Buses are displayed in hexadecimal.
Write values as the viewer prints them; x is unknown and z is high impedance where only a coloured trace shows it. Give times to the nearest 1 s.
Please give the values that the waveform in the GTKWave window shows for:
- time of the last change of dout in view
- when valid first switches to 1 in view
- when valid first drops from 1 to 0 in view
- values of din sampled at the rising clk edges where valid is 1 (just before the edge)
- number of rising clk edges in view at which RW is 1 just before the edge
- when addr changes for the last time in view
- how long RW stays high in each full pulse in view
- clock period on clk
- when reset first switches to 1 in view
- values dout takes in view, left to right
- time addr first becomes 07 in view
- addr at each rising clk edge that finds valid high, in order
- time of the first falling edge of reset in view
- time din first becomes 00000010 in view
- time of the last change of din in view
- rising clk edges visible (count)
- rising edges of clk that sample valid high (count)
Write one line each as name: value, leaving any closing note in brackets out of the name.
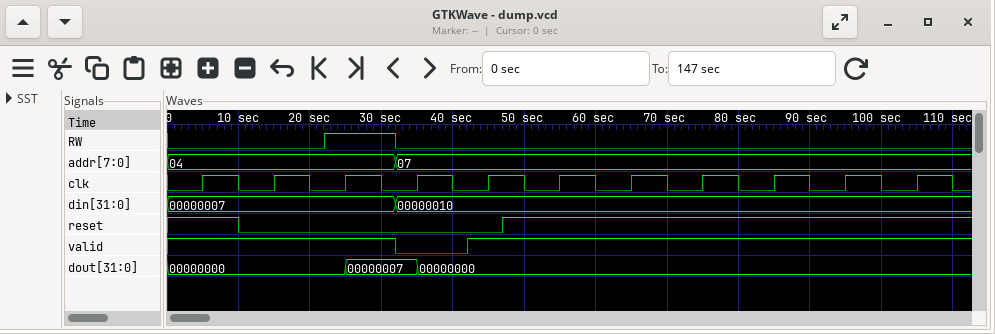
time of the last change of dout in view: 35 s
when valid first switches to 1 in view: 42 s
when valid first drops from 1 to 0 in view: 32 s
values of din sampled at the rising clk edges where valid is 1: 00000007, 00000007, 00000007, 00000010, 00000010, 00000010, 00000010, 00000010, 00000010, 00000010
number of rising clk edges in view at which RW is 1 just before the edge: 1
when addr changes for the last time in view: 32 s
how long RW stays high in each full pulse in view: 10 s
clock period on clk: 10 s
when reset first switches to 1 in view: 47 s
values dout takes in view, left to right: 00000000, 00000007, 00000000
time addr first becomes 07 in view: 32 s
addr at each rising clk edge that finds valid high, in order: 04, 04, 04, 07, 07, 07, 07, 07, 07, 07
time of the first falling edge of reset in view: 10 s
time din first becomes 00000010 in view: 32 s
time of the last change of din in view: 32 s
rising clk edges visible: 11
rising edges of clk that sample valid high: 10
